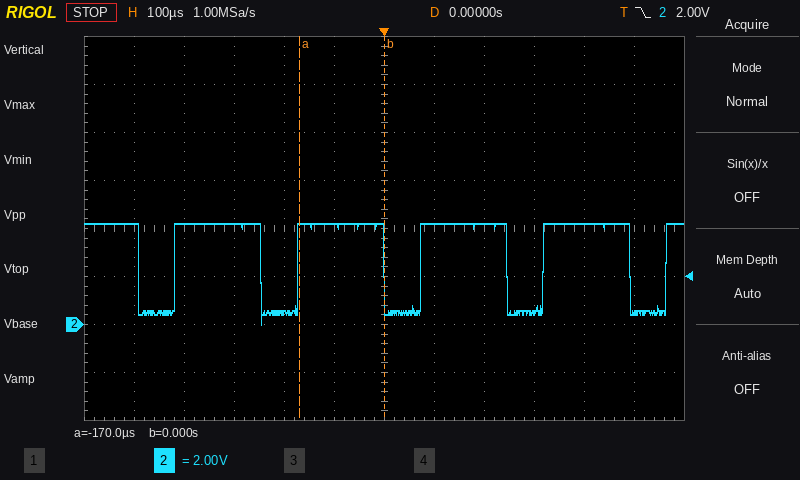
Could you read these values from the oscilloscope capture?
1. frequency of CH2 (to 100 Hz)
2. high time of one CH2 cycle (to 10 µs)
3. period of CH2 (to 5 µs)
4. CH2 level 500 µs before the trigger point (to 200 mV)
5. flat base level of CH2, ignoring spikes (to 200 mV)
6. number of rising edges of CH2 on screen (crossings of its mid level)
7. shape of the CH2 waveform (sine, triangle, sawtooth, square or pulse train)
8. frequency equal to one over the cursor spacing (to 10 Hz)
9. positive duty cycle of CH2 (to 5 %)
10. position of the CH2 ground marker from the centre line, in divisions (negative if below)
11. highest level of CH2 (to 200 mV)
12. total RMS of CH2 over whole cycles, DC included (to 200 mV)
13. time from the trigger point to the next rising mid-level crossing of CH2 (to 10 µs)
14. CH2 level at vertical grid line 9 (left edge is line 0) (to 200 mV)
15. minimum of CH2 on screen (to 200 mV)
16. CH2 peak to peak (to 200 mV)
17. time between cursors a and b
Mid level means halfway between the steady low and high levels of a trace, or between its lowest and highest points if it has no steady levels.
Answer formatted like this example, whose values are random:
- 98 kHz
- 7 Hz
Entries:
- 4.1 kHz
- 170 µs
- 245 µs
- 4.2 V
- 600 mV
- 5
- pulse train
- 5.88 kHz
- 70 %
- -2.0 div
- 4.2 V
- 3.6 V
- 70 µs
- 600 mV
- 0.0 V
- 4.2 V
- 170 µs
